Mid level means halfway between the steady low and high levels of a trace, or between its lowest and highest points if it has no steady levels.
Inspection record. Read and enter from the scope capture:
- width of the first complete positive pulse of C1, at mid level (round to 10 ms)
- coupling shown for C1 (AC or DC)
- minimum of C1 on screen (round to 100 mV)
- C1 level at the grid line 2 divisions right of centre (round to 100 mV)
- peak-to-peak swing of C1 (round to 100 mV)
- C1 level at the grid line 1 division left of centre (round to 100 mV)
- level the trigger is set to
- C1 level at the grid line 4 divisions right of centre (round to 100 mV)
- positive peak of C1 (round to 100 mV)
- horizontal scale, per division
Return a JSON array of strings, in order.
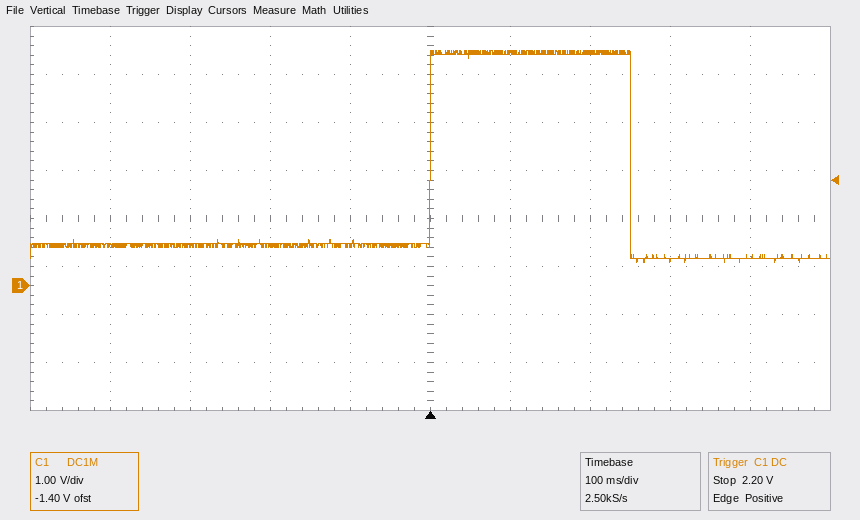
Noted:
["250 ms", "DC", "500 mV", "4.9 V", "4.4 V", "900 mV", "2.20 V", "600 mV", "4.9 V", "100 ms"]
